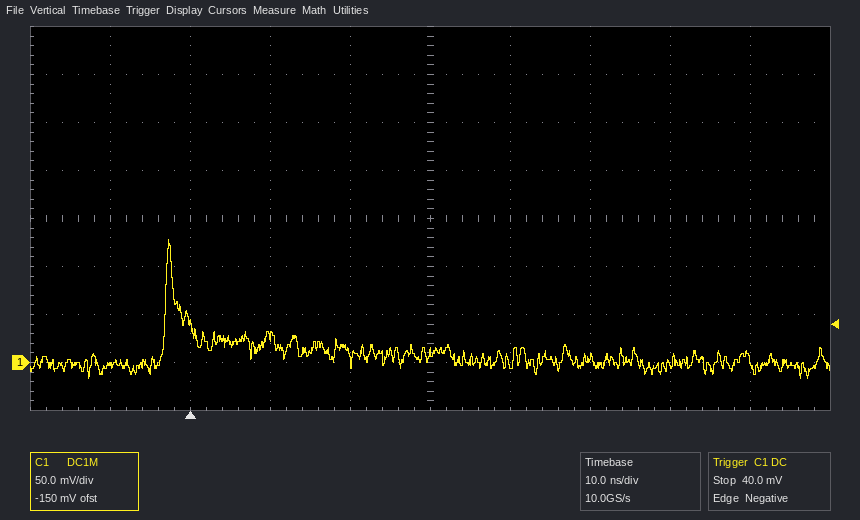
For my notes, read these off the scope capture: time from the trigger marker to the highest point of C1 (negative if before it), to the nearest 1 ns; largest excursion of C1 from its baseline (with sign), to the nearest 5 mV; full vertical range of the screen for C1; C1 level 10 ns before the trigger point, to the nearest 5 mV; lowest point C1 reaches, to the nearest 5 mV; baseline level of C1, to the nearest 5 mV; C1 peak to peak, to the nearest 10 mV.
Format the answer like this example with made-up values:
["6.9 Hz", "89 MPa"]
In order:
["-3 ns", "+125 mV", "400 mV", "-5 mV", "-15 mV", "0 mV", "140 mV"]
